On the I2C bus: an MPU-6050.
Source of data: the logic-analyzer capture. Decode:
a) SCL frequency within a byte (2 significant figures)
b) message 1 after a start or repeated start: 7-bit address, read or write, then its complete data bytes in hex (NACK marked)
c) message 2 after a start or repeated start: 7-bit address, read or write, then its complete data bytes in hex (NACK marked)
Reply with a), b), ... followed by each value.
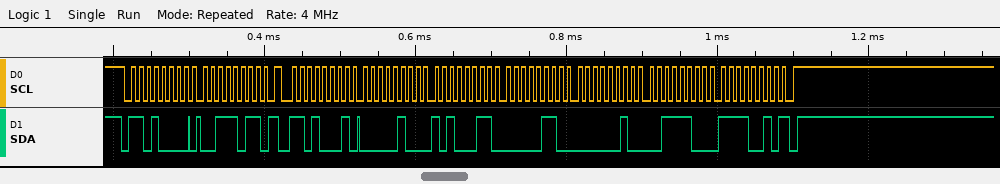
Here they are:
a) 100 kHz
b) 0x68 write: 3B
c) 0x68 read: 04 A3 06 02 3C F2 NACK
